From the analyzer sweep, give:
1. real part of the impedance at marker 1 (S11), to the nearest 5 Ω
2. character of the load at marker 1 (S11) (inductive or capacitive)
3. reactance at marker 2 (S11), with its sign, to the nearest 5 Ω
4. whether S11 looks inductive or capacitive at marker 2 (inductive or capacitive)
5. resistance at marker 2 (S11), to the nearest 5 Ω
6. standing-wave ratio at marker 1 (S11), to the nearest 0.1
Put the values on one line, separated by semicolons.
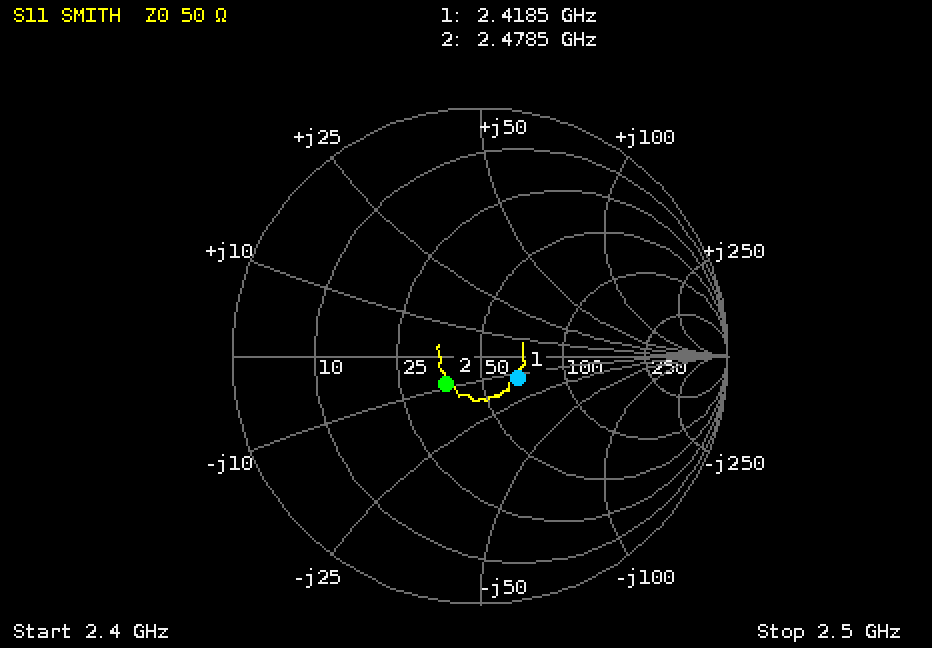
65 Ω; capacitive; -10 Ω; capacitive; 35 Ω; 1.4
